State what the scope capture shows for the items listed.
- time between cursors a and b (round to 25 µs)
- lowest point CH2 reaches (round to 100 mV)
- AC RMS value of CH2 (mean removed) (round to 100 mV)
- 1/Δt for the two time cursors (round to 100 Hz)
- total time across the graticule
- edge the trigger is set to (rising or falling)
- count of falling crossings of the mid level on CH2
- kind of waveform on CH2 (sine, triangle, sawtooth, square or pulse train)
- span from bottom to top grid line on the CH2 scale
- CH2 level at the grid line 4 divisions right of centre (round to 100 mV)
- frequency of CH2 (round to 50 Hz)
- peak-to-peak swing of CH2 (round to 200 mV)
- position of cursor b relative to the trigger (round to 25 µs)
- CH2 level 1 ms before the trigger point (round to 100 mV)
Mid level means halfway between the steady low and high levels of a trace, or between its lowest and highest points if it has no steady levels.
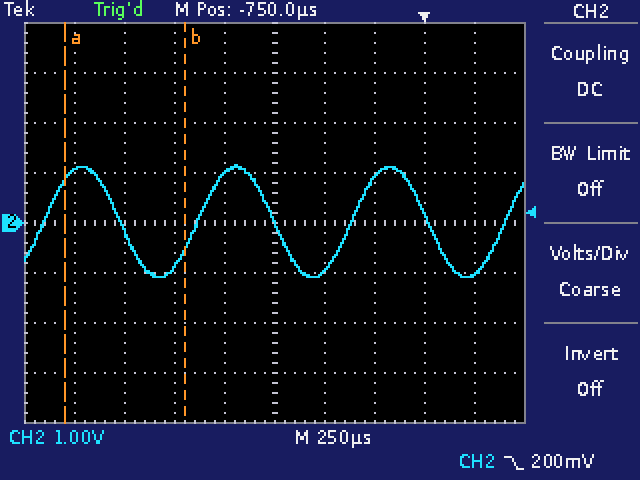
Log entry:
600 µs
-1.1 V
800 mV
1.7 kHz
2.5 ms
falling
3
sine
8 V
-1.0 V
1.30 kHz
2.2 V
-1.200 ms
1.0 V
